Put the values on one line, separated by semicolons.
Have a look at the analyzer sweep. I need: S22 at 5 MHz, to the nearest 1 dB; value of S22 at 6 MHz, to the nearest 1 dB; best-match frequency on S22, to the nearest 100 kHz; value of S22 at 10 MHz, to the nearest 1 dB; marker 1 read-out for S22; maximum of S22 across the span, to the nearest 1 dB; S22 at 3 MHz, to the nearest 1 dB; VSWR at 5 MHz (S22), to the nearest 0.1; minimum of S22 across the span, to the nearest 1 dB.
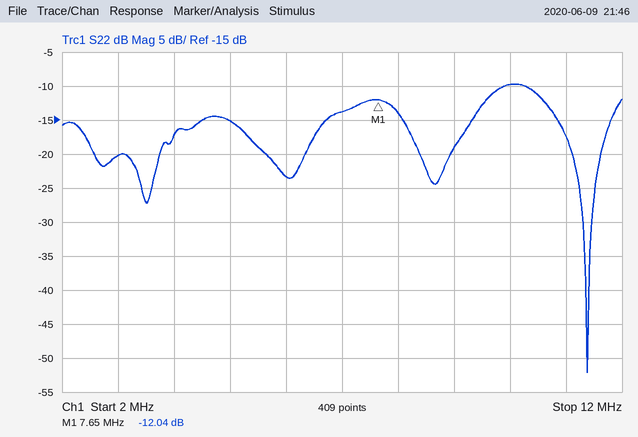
-15 dB; -23 dB; 11.4 MHz; -10 dB; -12.04 dB; -10 dB; -20 dB; 1.4; -52 dB
